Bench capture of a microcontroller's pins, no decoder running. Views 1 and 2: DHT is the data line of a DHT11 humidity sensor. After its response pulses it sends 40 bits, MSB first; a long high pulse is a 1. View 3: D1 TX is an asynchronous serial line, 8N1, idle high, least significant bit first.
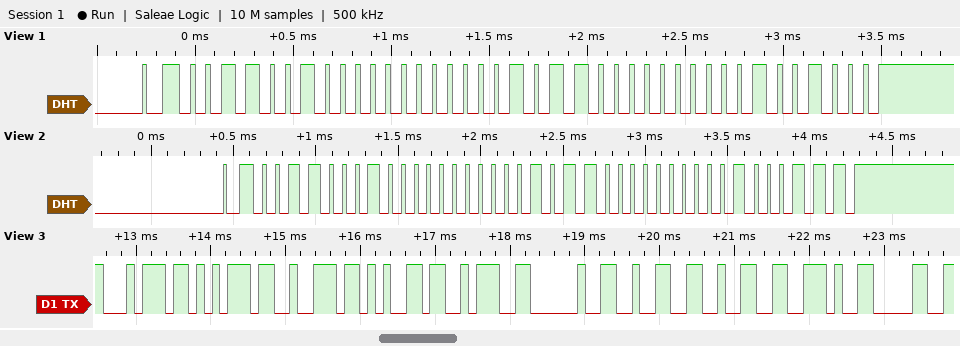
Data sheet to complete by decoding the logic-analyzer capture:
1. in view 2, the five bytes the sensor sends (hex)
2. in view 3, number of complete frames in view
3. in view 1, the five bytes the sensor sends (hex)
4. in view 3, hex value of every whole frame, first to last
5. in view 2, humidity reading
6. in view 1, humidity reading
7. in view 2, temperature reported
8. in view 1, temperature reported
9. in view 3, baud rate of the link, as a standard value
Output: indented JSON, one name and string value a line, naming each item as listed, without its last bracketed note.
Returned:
{
  "in view 2, the five bytes the sensor sends": "31 00 16 00 47",
  "in view 3, number of complete frames in view": "10",
  "in view 1, the five bytes the sensor sends": "32 00 16 00 48",
  "in view 3, hex value of every whole frame, first to last": "74 75 72 65 3A 20 32 32 2E 30",
  "in view 2, humidity reading": "49 %",
  "in view 1, humidity reading": "50 %",
  "in view 2, temperature reported": "22.0 °C",
  "in view 1, temperature reported": "22.0 °C",
  "in view 3, baud rate of the link, as a standard value": "9600 baud"
}
